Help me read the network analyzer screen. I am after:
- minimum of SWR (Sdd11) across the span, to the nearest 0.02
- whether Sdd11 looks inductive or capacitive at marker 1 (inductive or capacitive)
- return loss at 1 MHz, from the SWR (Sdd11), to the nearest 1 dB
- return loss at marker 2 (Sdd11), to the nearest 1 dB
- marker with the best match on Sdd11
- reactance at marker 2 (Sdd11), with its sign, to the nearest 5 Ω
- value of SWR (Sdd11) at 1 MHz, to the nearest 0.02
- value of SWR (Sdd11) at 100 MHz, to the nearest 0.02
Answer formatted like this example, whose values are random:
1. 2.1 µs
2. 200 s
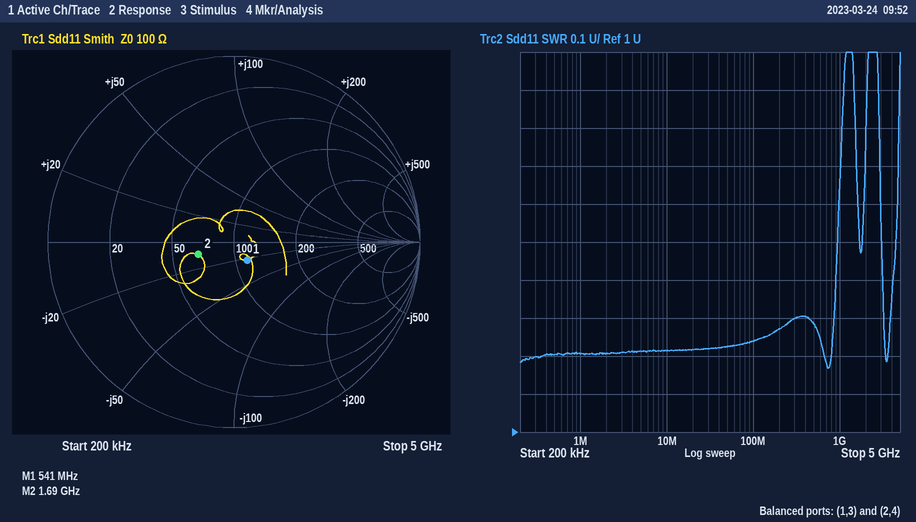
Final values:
1. 1.16
2. capacitive
3. 21 dB
4. 14 dB
5. marker 1
6. -10 Ω
7. 1.20
8. 1.24
